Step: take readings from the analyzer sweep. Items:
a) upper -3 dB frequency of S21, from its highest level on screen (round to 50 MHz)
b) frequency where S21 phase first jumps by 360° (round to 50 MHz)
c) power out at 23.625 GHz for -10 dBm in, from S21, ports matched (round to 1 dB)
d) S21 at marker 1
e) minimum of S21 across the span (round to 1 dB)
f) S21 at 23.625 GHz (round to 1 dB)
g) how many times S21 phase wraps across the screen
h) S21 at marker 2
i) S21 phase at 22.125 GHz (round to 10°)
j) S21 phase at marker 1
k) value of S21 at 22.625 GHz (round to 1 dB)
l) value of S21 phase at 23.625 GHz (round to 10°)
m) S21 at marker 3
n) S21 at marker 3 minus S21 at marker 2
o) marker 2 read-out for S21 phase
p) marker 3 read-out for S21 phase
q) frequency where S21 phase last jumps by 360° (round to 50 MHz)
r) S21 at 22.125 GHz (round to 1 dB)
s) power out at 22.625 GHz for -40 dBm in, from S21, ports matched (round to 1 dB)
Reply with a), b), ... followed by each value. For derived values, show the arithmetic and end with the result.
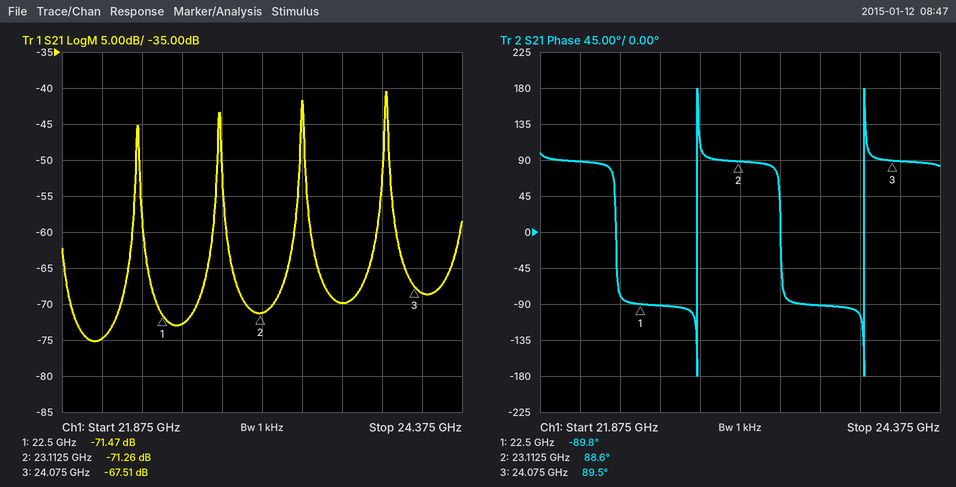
a) 23.90 GHz
b) 22.85 GHz
c) -10 dBm + (-70 dB) = -80 dBm
d) -71.47 dB
e) -75 dB
f) -70 dB
g) 2
h) -71.26 dB
i) 90°
j) -89.8°
k) -73 dB
l) -90°
m) -67.51 dB
n) -67.51 − (-71.26) = 3.75 dB
o) 88.6°
p) 89.5°
q) 23.90 GHz
r) -75 dB
s) -40 dBm + (-73 dB) = -113 dBm
